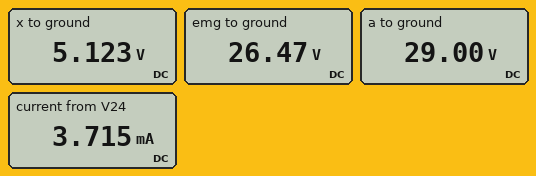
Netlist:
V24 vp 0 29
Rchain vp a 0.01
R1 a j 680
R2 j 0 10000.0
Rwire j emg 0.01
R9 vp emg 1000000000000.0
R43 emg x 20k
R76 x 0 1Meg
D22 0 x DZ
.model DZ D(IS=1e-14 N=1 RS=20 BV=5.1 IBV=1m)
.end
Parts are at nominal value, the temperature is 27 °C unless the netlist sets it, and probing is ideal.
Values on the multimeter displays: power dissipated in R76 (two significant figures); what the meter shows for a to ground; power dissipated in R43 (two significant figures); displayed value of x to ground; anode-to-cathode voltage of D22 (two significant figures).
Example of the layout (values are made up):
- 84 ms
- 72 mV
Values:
- 26 µW
- 29.00 V
- 23 mW
- 5.123 V
- -5.1 V
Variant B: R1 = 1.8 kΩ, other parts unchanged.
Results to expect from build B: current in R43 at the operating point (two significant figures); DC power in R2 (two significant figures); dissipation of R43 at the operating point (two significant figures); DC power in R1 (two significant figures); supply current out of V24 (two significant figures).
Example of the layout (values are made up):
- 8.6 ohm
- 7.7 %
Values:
- 900 µA
- 54 mW
- 16 mW
- 19 mW
- 3.2 mA
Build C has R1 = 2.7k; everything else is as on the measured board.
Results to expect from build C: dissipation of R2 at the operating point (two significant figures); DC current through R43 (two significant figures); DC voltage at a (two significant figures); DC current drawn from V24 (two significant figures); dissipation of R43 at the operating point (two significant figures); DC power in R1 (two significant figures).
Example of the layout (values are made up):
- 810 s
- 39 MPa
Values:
- 45 mW
- 800 µA
- 29 V
- 2.9 mA
- 13 mW
- 23 mW
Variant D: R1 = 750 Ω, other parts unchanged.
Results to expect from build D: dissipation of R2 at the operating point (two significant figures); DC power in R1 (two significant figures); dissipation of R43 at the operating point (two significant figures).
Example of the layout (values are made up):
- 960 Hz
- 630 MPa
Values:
- 69 mW
- 10 mW
- 22 mW
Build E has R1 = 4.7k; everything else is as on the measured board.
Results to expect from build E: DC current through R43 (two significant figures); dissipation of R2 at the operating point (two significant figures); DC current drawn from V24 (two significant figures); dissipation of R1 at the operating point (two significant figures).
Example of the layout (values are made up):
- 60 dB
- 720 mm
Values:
- 630 µA
- 31 mW
- 2.4 mA
- 27 mW
